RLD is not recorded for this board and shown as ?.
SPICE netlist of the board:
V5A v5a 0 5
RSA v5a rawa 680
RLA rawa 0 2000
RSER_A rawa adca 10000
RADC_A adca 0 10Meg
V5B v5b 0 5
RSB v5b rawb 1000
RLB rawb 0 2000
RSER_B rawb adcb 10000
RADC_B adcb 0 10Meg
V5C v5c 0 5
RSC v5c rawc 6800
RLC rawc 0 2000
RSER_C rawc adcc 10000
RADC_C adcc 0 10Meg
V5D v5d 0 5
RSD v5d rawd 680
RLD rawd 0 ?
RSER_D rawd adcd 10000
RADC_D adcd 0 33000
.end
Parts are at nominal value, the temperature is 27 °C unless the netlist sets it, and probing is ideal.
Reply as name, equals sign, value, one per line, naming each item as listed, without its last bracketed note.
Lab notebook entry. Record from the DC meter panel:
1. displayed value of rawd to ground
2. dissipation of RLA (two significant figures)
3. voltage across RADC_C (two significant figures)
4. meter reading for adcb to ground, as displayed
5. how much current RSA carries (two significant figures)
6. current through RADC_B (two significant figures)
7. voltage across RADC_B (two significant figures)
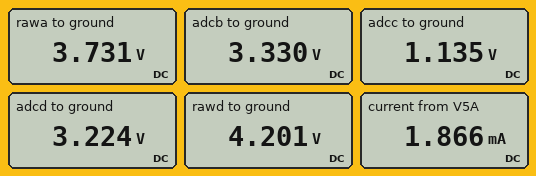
displayed value of rawd to ground = 4.201 V
dissipation of RLA = 7.0 mW
voltage across RADC_C = 1.1 V
meter reading for adcb to ground, as displayed = 3.330 V
how much current RSA carries = 1.9 mA
current through RADC_B = 330 nA
voltage across RADC_B = 3.3 V
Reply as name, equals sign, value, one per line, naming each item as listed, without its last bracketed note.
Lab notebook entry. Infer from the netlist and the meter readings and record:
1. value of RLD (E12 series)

value of RLD = 3.9 kΩ
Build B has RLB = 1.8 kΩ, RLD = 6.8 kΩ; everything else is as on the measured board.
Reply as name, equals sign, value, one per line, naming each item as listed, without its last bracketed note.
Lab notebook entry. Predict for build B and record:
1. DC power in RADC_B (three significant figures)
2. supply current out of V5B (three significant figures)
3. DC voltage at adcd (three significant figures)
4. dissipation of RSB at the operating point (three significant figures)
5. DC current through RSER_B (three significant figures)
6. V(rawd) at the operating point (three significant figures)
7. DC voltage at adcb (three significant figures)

DC power in RADC_B = 1.03 µW
supply current out of V5B = 1.79 mA
DC voltage at adcd = 3.44 V
dissipation of RSB at the operating point = 3.19 mW
DC current through RSER_B = 321 nA
V(rawd) at the operating point = 4.48 V
DC voltage at adcb = 3.21 V
